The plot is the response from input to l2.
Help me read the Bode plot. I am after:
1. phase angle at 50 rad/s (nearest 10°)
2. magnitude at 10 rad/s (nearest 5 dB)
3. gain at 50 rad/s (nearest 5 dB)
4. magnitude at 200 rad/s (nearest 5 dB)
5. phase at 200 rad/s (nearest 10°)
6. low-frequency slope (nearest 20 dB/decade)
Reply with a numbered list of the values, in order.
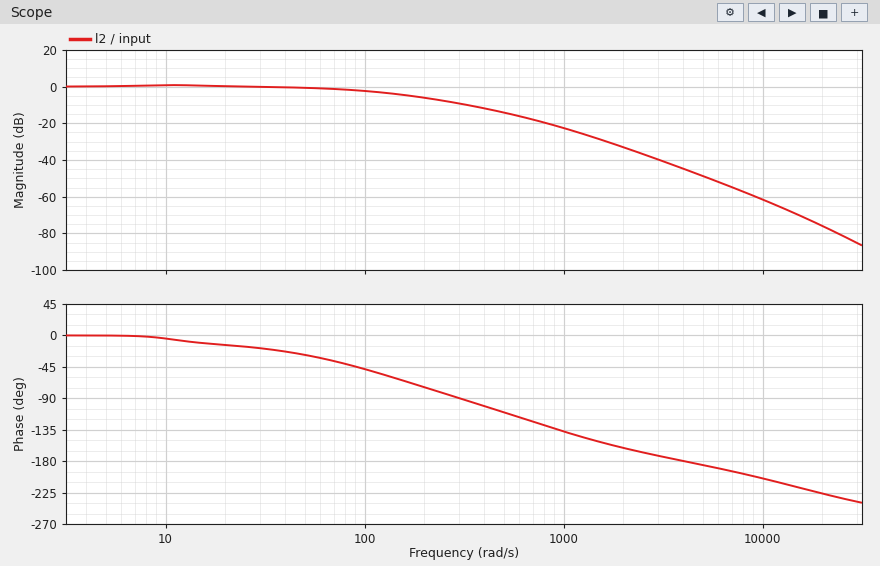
1. -30°
2. 0 dB
3. 0 dB
4. -5 dB
5. -70°
6. 0 dB/decade
